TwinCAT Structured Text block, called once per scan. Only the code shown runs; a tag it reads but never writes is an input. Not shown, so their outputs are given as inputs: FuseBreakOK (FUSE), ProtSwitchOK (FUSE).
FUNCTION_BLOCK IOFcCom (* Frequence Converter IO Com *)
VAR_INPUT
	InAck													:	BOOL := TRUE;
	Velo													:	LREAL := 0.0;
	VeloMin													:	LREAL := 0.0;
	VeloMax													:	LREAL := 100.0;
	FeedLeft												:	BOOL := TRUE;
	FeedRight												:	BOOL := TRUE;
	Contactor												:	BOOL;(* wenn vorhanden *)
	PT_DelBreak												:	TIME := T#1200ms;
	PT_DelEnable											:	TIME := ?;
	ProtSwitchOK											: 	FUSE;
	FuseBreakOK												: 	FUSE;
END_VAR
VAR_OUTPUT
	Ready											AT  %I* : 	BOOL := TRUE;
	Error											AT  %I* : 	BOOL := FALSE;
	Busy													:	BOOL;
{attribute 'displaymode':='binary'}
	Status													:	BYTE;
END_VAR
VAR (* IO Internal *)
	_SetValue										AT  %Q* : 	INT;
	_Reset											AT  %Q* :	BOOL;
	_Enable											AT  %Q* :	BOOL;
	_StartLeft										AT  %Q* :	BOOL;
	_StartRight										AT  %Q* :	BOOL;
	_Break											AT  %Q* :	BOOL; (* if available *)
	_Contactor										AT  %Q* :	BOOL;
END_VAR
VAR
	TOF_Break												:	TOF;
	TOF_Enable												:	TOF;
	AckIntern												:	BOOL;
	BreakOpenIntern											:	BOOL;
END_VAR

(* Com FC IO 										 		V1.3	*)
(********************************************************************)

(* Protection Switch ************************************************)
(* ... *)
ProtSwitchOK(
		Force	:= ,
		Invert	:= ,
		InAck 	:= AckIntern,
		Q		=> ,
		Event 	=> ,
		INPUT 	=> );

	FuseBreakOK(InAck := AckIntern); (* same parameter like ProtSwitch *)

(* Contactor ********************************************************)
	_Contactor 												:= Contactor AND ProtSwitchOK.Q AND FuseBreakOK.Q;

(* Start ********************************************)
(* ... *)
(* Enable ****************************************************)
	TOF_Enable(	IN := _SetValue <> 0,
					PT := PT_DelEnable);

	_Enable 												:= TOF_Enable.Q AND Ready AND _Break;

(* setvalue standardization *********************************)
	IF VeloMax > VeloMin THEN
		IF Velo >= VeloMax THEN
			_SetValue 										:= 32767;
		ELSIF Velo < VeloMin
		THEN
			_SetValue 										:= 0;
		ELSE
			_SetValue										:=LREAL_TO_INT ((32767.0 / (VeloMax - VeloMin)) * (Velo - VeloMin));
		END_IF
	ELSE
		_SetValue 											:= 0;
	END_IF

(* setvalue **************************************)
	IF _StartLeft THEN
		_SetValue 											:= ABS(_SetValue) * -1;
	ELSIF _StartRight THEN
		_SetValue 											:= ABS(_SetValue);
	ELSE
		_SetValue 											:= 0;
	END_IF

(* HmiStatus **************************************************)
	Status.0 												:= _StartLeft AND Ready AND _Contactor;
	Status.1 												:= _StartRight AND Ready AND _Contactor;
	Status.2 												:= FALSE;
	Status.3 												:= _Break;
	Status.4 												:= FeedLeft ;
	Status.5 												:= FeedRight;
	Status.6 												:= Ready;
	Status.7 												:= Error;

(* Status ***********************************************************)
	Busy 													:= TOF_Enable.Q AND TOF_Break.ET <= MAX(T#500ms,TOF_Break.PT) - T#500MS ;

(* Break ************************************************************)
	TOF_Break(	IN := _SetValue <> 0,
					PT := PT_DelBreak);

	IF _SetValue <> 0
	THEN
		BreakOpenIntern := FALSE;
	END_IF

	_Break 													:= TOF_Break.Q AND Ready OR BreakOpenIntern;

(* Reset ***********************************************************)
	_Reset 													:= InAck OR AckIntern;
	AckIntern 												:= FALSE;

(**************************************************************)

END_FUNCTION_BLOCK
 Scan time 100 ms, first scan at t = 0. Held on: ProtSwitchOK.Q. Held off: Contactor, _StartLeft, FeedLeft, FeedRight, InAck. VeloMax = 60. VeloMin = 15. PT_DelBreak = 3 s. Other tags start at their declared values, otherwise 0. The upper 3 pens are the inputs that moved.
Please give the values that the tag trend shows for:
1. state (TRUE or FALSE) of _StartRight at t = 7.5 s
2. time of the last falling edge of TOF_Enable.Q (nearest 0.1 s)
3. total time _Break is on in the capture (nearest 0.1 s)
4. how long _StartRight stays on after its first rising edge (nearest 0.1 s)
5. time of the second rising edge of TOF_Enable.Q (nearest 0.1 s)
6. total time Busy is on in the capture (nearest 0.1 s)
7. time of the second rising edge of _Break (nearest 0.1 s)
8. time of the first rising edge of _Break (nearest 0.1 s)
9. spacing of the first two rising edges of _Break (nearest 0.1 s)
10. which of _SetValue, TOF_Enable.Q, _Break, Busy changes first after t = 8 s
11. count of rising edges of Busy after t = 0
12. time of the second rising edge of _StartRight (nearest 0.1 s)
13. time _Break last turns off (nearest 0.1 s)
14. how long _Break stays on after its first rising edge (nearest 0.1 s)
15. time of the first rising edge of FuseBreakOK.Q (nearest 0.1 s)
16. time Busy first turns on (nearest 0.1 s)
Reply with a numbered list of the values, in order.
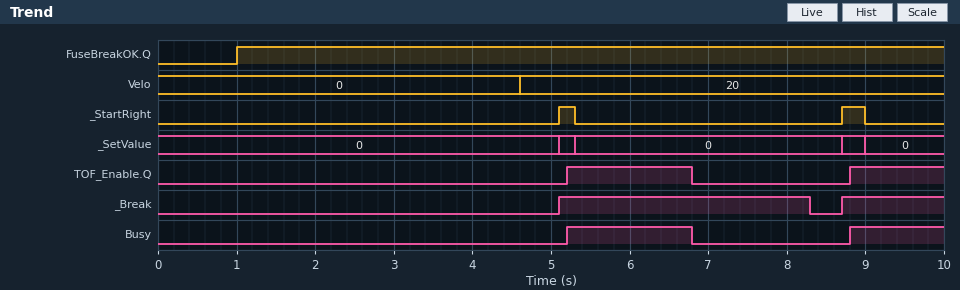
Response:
1. FALSE
2. 6.8 s
3. 4.5 s
4. 0.2 s
5. 8.8 s
6. 2.8 s
7. 8.7 s
8. 5.1 s
9. 3.6 s
10. _Break
11. 2
12. 8.7 s
13. 8.3 s
14. 3.2 s
15. 1.0 s
16. 5.2 s
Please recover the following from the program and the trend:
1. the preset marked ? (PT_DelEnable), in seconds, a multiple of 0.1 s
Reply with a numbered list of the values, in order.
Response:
1. 1.4 s
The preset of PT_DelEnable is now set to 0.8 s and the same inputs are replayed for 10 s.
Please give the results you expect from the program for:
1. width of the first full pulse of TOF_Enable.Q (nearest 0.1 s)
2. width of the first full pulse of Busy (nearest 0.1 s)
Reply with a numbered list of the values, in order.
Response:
1. 1.0 s
2. 1.0 s
